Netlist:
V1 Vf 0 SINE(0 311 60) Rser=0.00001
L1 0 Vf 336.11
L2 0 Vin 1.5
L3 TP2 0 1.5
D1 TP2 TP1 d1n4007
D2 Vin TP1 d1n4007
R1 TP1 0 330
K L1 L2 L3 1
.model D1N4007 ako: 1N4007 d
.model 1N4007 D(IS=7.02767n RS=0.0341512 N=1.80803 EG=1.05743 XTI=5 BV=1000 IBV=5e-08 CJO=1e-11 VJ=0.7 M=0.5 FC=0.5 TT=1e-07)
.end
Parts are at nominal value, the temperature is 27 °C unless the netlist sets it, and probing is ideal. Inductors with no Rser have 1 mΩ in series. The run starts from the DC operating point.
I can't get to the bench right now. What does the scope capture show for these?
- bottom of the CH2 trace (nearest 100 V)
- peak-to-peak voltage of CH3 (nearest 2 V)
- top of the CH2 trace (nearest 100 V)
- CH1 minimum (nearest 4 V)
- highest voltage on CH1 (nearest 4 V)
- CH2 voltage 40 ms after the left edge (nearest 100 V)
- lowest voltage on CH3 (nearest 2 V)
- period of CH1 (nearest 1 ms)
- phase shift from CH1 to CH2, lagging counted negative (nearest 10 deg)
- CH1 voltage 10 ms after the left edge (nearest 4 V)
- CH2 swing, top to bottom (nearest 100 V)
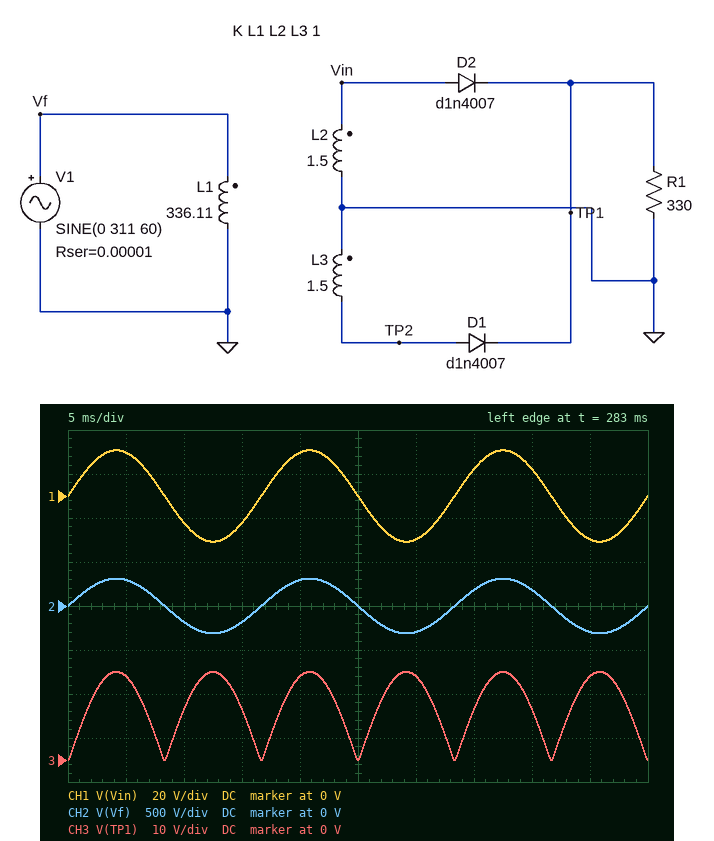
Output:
-300 V
20 V
300 V
-20 V
20 V
200 V
0 V
17 ms
0 deg
-12 V
600 V
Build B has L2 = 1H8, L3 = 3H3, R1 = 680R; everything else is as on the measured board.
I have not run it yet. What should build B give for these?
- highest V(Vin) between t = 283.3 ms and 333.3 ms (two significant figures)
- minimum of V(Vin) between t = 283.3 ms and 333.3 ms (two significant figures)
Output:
23 V
-23 V
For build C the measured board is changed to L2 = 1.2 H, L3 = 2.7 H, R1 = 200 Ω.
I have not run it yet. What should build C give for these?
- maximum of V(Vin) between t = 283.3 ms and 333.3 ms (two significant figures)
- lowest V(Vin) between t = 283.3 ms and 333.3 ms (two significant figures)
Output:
19 V
-19 V
